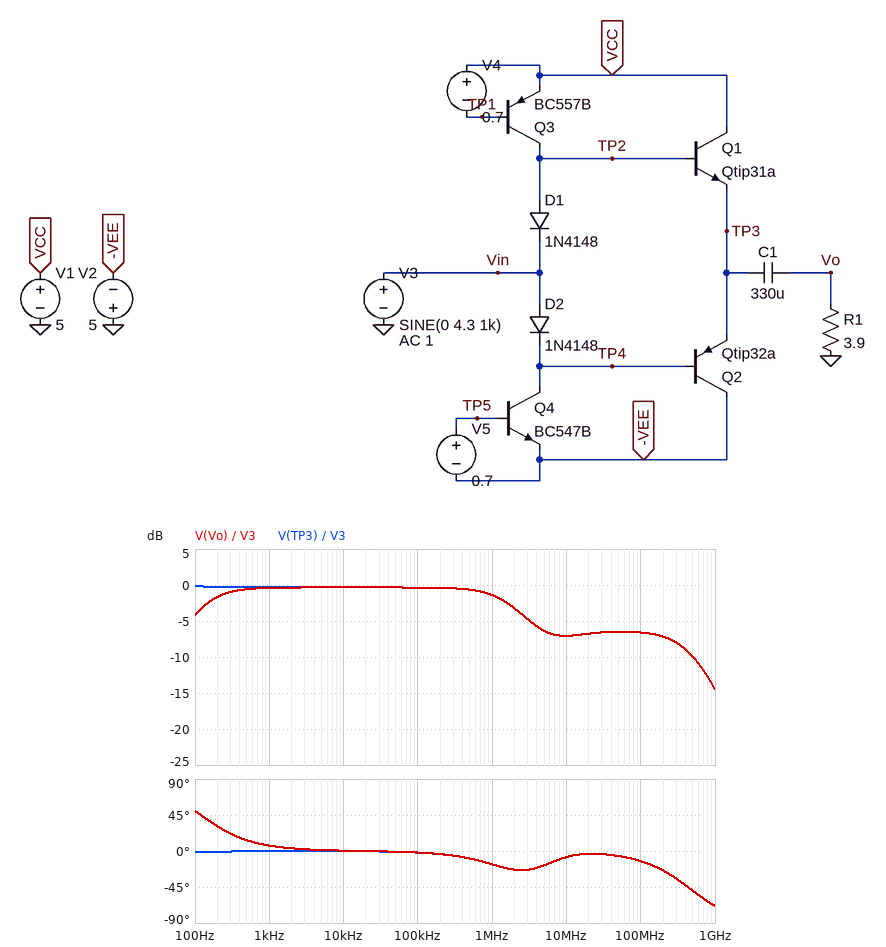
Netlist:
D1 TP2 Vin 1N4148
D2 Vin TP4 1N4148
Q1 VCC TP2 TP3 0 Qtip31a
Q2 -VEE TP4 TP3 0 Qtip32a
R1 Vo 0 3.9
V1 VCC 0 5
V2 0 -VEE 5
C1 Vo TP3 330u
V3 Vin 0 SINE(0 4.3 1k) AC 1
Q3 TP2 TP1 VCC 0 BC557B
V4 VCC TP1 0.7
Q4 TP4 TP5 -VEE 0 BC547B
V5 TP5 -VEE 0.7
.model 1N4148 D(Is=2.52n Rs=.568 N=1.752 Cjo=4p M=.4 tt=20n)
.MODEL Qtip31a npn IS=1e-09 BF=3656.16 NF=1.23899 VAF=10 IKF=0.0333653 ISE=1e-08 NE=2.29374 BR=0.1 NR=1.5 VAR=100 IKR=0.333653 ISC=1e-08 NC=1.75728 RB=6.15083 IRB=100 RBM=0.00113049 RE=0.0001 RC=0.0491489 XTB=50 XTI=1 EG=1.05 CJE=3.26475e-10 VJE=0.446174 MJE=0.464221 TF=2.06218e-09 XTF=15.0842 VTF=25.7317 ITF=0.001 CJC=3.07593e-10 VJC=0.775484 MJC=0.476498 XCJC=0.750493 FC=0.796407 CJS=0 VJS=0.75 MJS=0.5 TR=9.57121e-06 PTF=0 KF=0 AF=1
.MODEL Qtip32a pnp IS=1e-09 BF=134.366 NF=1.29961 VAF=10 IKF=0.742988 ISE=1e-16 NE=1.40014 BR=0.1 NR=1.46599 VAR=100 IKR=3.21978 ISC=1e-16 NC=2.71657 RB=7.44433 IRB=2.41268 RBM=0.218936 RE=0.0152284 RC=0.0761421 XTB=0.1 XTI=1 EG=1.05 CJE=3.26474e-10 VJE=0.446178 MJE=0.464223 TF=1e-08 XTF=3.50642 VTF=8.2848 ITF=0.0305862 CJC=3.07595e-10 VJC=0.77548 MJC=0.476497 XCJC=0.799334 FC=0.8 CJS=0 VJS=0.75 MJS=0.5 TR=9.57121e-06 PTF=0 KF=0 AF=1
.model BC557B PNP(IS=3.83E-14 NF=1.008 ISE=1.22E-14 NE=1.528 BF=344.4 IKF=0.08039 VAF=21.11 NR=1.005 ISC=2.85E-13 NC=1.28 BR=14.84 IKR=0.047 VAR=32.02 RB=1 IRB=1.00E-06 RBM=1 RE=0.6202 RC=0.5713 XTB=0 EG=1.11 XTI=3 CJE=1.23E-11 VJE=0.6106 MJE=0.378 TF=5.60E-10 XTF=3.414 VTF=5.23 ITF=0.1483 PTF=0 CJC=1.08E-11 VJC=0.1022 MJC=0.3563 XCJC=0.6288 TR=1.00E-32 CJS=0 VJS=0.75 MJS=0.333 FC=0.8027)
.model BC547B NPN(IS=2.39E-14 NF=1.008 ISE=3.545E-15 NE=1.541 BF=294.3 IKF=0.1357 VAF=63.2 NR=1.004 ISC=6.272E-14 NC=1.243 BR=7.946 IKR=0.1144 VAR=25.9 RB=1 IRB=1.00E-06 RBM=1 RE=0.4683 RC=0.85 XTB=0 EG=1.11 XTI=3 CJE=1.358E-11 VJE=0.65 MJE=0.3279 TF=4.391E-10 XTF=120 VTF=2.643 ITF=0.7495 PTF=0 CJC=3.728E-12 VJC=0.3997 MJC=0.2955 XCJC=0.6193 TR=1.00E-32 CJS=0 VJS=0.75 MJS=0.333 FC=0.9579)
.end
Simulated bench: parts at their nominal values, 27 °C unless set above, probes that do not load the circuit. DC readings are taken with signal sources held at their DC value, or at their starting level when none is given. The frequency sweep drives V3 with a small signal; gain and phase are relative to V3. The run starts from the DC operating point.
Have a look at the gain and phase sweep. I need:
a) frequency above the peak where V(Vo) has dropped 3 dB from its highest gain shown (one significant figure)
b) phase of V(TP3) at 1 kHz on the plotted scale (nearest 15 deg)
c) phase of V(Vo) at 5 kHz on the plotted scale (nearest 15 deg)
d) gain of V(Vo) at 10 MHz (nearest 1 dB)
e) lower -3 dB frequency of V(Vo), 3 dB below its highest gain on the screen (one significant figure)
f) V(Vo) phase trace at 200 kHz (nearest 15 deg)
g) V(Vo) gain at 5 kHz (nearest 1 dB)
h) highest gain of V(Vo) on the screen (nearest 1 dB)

2 MHz
0 deg
0 deg
-7 dB
100 Hz
0 deg
0 dB
0 dB
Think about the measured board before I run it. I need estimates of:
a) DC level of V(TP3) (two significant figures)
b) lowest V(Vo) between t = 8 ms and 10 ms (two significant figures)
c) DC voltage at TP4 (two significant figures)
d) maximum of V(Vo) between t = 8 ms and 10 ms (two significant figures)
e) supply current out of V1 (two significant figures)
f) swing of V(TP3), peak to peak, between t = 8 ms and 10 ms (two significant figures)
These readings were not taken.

6.0 mV
-2.9 V
-670 mV
3.6 V
350 mA
6.8 V
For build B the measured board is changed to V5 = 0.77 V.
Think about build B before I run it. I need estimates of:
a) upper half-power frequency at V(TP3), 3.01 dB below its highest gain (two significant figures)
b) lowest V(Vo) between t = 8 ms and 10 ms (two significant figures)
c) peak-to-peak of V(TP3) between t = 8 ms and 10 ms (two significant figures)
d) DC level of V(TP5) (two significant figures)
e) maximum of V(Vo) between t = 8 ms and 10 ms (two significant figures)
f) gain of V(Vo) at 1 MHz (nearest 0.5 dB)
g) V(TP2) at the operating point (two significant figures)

2.2 MHz
-4.0 V
7.9 V
-4.2 V
3.8 V
-1.0 dB
690 mV
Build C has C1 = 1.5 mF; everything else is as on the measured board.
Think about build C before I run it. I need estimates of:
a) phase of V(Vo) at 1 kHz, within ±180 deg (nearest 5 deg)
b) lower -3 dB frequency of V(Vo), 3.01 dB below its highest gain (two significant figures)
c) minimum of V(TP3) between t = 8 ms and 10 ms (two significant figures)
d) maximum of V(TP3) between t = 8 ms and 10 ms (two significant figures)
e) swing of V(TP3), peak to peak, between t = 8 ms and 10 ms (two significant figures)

0 deg
26 Hz
-2.7 V
3.9 V
6.6 V
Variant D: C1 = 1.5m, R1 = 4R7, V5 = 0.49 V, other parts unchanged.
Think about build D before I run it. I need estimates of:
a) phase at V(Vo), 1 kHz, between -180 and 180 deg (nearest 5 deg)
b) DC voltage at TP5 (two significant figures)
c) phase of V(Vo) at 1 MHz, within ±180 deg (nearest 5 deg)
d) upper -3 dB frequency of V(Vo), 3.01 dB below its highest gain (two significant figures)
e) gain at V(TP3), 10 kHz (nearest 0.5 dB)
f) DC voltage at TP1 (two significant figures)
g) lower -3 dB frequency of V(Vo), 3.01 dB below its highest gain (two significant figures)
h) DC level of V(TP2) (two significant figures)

0 deg
-4.5 V
10 deg
310 MHz
-20.5 dB
4.3 V
14 MHz
710 mV
